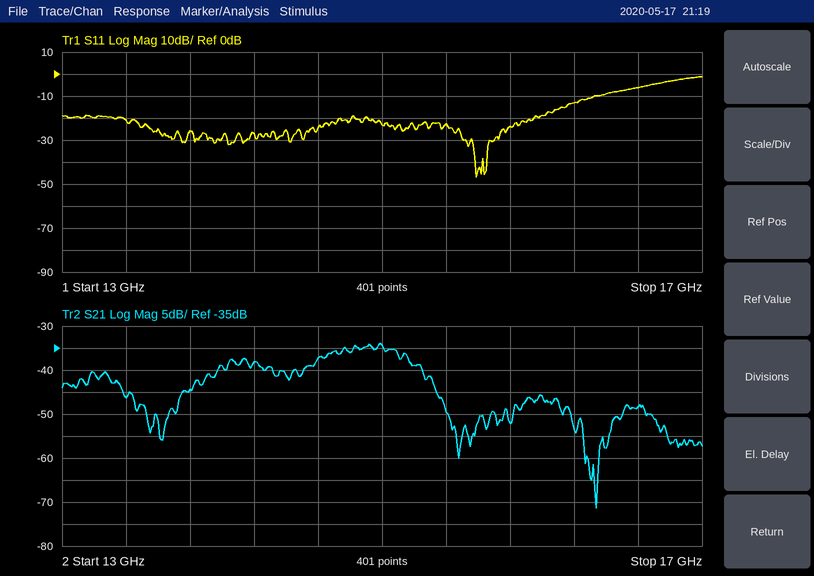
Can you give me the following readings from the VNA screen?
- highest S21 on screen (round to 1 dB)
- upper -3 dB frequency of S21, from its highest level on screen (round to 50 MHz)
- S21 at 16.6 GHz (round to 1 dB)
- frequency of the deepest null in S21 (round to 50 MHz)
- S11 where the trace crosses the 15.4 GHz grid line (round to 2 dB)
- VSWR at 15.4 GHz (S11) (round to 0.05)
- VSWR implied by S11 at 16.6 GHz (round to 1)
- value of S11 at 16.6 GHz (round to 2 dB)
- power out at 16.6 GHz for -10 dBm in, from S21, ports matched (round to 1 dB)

-34 dB
15.10 GHz
-48 dB
16.35 GHz
-22 dB
1.15
3
-6 dB
-58 dBm
